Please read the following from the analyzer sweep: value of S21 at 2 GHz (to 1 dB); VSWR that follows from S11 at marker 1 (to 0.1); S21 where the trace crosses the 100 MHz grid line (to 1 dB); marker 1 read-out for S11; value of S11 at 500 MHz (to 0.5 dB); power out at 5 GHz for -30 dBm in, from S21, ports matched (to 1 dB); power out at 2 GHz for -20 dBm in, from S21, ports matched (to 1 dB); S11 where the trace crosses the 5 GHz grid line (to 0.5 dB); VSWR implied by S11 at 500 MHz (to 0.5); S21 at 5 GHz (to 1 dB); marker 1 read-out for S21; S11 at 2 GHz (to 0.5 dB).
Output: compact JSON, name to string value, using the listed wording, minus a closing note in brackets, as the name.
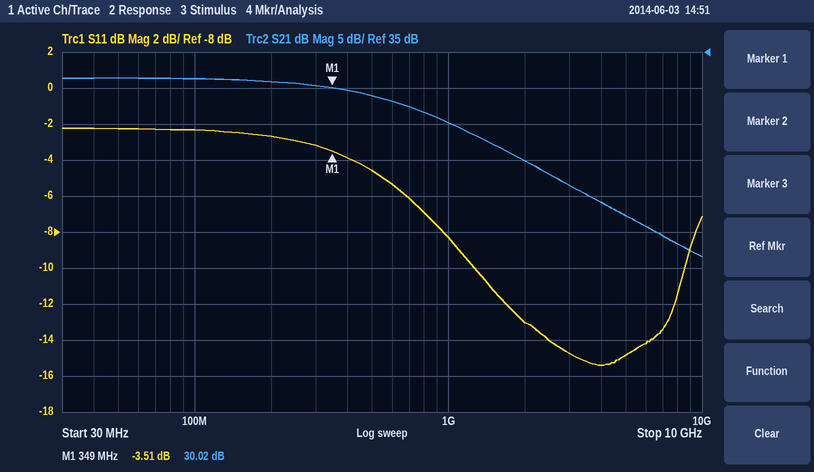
{"value of S21 at 2 GHz": "20 dB", "VSWR that follows from S11 at marker 1": "5.0", "S21 where the trace crosses the 100 MHz grid line": "31 dB", "marker 1 read-out for S11": "-3.51 dB", "value of S11 at 500 MHz": "-4.5 dB", "power out at 5 GHz for -30 dBm in, from S21, ports matched": "-18 dBm", "power out at 2 GHz for -20 dBm in, from S21, ports matched": "0 dBm", "S11 where the trace crosses the 5 GHz grid line": "-15.0 dB", "VSWR implied by S11 at 500 MHz": "4.0", "S21 at 5 GHz": "12 dB", "marker 1 read-out for S21": "30.02 dB", "S11 at 2 GHz": "-13.0 dB"}
